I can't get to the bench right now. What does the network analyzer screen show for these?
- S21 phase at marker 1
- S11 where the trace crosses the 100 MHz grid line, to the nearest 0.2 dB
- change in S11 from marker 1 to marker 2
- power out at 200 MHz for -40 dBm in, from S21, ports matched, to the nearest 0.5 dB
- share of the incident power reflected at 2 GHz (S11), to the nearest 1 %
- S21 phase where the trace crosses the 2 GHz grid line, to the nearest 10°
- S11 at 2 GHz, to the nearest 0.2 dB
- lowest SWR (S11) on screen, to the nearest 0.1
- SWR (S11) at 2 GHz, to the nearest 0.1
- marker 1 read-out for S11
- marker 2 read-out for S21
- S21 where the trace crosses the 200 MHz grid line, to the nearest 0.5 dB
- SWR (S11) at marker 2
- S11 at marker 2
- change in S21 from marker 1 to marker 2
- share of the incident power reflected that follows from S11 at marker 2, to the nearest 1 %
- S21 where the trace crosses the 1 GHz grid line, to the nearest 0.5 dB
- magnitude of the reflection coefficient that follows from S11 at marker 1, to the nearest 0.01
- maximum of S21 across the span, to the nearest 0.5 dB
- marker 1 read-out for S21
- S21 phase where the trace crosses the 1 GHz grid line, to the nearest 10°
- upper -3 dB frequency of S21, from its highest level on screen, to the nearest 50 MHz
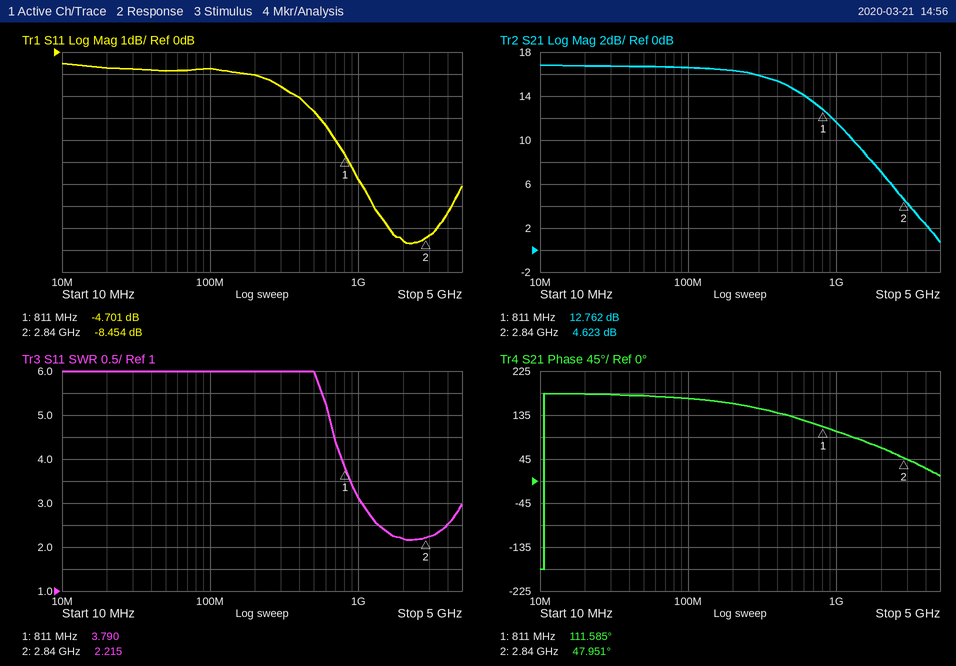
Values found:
111.585°
-0.8 dB
-3.753 dB
-23.5 dBm
14 %
70°
-8.6 dB
2.2
2.2
-4.701 dB
4.623 dB
16.5 dB
2.215
-8.454 dB
-8.139 dB
14 %
11.5 dB
0.58
17.0 dB
12.762 dB
100°
650 MHz
